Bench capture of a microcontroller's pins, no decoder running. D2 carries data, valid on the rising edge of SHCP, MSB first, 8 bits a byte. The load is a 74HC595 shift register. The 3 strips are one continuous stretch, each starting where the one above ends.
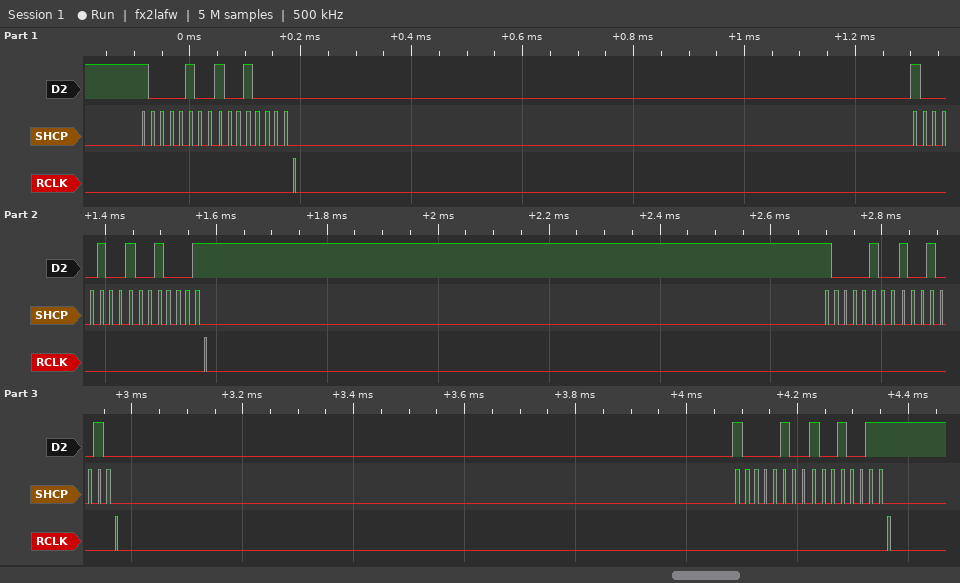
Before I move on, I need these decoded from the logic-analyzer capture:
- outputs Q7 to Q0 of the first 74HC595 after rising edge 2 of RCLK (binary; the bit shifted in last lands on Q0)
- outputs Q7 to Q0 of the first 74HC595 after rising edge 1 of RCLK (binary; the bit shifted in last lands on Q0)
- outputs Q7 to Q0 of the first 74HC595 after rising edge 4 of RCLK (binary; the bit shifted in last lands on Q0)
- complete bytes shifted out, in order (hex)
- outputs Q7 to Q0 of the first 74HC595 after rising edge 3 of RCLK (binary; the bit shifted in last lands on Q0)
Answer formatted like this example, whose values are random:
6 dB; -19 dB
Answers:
10010001; 10010000; 10010011; 0x84 0x90 0x84 0x91 0x84 0x92 0x84 0x93; 10010010
